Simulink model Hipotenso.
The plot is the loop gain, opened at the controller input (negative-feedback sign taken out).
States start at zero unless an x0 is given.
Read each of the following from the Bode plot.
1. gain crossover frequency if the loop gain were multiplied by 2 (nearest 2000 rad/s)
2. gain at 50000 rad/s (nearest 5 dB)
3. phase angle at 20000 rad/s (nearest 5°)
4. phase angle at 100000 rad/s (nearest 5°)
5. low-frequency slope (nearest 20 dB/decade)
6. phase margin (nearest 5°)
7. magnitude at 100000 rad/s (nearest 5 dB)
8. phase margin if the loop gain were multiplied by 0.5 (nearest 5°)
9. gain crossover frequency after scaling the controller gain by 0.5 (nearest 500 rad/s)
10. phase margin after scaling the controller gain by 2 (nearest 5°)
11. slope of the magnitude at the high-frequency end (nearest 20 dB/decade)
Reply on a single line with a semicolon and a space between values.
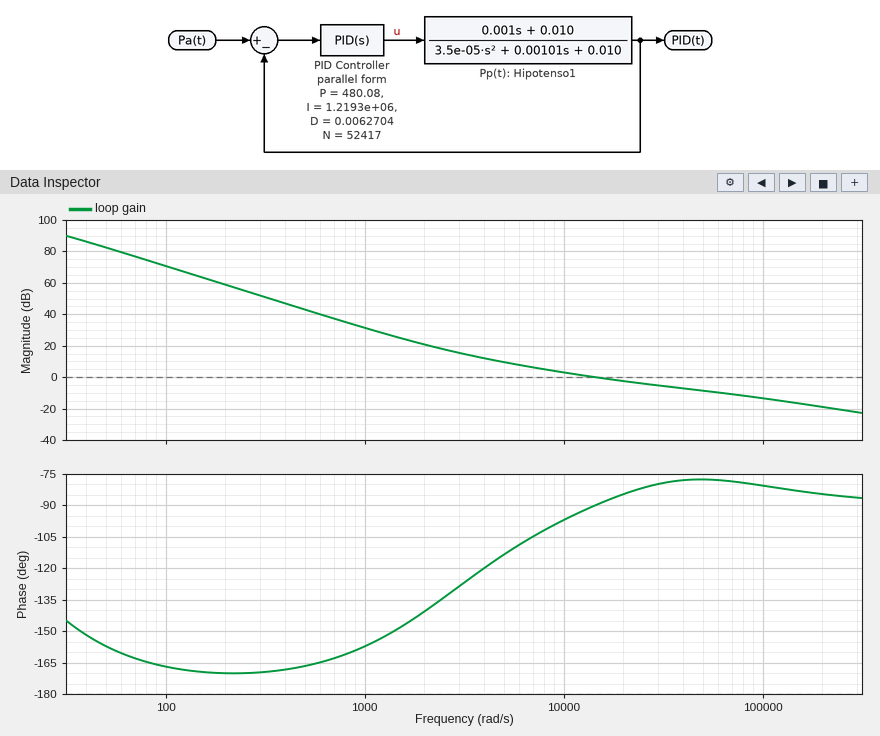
34000 rad/s; -10 dB; -85°; -80°; -40 dB/decade; 90°; -15 dB; 75°; 7000 rad/s; 100°; -20 dB/decade
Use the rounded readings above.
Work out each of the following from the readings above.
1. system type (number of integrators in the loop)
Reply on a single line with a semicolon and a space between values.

2
